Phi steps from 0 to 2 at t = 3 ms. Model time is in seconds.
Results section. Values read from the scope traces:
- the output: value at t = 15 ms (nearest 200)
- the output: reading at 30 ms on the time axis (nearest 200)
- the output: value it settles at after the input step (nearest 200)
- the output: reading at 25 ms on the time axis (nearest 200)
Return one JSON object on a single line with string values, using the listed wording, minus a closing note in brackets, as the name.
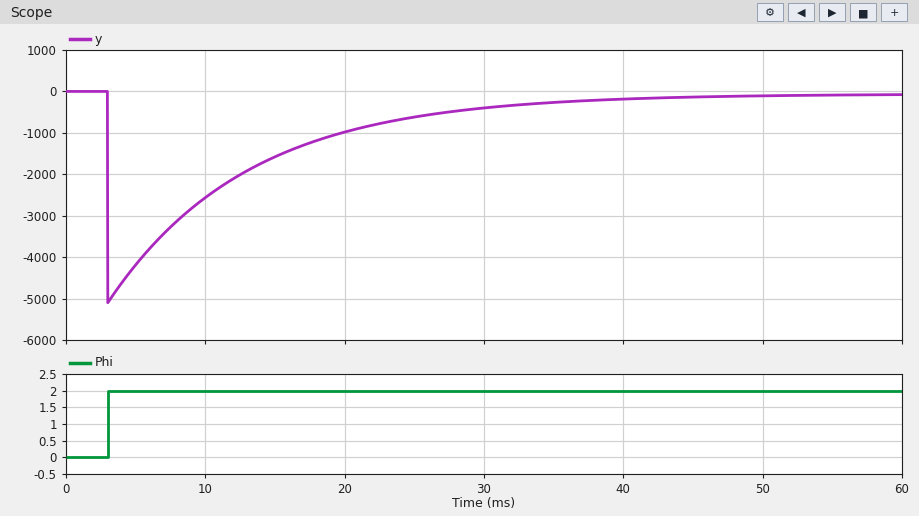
{"the output: value at t = 15 ms": "-1600", "the output: reading at 30 ms on the time axis": "-400", "the output: value it settles at after the input step": "0", "the output: reading at 25 ms on the time axis": "-600"}
